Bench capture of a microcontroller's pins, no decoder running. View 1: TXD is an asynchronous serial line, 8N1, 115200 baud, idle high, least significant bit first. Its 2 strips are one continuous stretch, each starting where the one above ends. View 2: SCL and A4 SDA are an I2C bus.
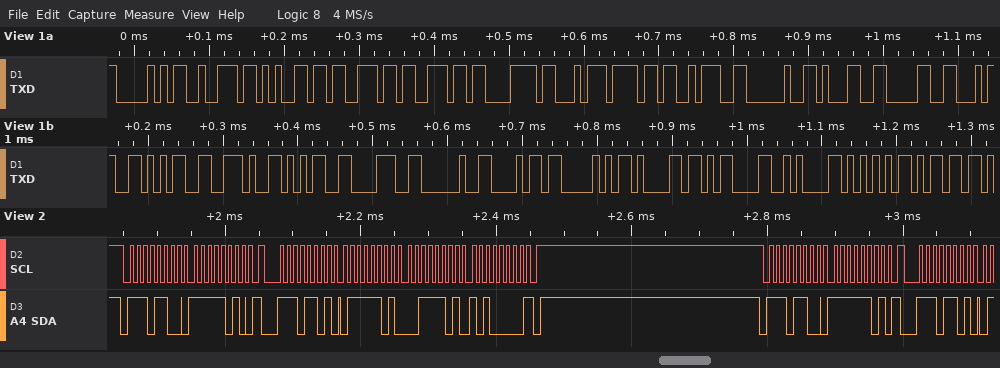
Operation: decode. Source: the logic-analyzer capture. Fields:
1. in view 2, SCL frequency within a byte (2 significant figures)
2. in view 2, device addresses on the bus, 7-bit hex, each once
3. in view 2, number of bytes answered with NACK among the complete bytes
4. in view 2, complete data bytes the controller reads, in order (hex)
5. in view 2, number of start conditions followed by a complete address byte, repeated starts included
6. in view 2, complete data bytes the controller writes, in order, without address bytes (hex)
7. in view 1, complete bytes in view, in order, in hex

100 kHz
0x76
1
7D 3D A0
4
FA FD
0x50 0x72 0x65 0x73 0x73 0xC3 0xA3 0x6F 0x3A 0x20 0x31 0x30 0x34 0x35 0x2E 0x35 0x38 0x20 0x68 0x50 0x61 0x0D 0x0A 0x55 0x6D
